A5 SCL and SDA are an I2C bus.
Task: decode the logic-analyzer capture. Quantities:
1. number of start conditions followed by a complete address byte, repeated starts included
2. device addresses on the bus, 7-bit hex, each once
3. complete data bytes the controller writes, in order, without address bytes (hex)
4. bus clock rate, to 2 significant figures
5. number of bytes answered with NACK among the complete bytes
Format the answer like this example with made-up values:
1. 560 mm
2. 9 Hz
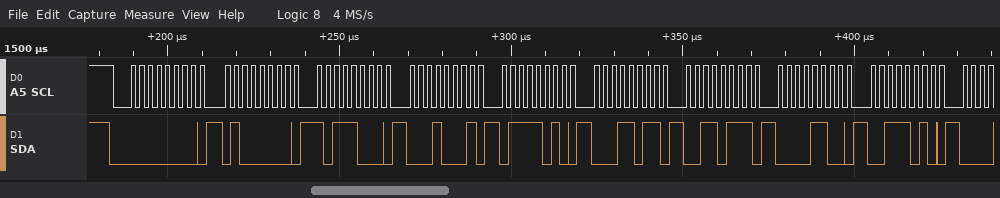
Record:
1. 1
2. 0x00
3. 40 B8 11 7A 1B 37 0C 3A
4. 400 kHz
5. 0
